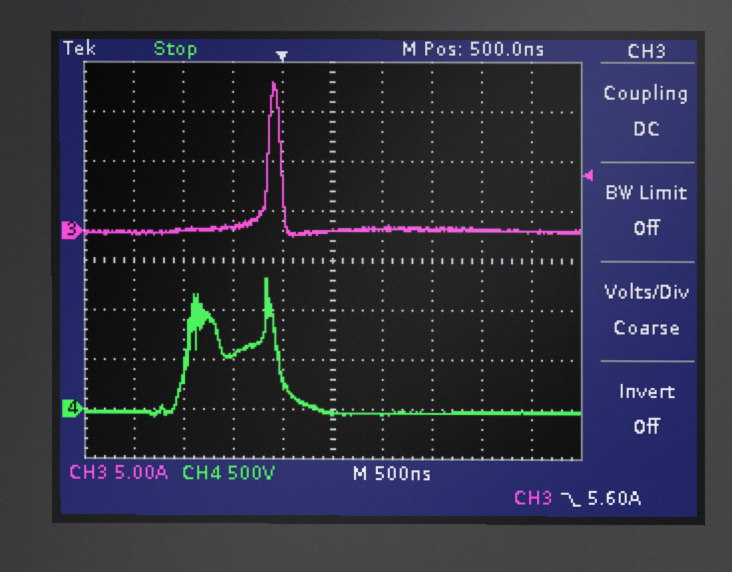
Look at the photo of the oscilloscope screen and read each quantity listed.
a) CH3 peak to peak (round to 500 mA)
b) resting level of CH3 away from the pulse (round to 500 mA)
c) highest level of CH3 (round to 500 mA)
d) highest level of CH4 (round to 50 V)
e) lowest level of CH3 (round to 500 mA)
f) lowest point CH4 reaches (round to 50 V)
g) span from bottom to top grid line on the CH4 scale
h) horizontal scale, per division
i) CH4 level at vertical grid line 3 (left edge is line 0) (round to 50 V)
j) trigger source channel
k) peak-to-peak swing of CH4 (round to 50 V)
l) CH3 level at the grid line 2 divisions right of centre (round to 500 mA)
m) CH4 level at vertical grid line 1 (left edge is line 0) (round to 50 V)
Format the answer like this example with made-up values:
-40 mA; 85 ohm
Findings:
15.5 A; 0.0 A; 15.0 A; 1.30 kV; -500 mA; -100 V; 4 kV; 500 ns; 550 V; CH3; 1.40 kV; 0.0 A; -50 V
